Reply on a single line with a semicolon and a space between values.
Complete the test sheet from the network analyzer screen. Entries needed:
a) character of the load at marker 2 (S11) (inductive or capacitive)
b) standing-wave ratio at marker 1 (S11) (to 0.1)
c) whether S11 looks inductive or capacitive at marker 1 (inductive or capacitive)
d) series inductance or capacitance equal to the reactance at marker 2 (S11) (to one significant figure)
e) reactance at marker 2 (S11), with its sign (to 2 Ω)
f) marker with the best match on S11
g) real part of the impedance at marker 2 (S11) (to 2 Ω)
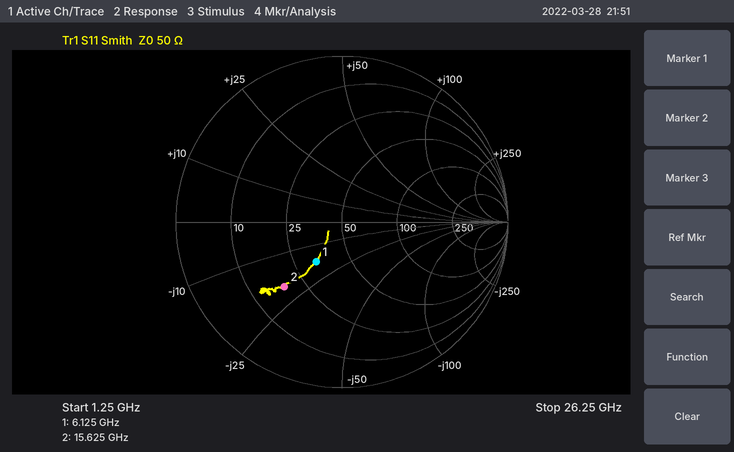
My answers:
capacitive; 1.8; capacitive; 500 fF; -20 Ω; marker 1; 18 Ω
